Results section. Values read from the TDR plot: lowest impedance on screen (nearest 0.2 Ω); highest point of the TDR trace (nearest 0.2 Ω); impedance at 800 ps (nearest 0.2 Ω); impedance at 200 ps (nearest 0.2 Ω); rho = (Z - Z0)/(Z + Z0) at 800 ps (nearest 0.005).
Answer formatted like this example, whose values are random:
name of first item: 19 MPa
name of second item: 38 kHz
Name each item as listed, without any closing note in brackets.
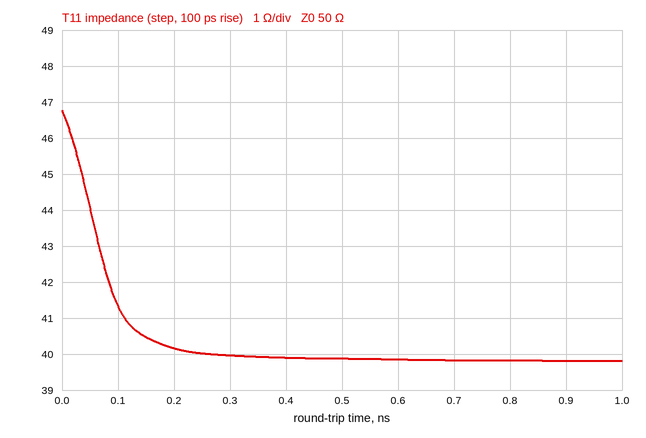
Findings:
lowest impedance on screen: 39.8 Ω
highest point of the TDR trace: 46.8 Ω
impedance at 800 ps: 39.8 Ω
impedance at 200 ps: 40.2 Ω
rho = (Z - Z0)/(Z + Z0) at 800 ps: -0.115
